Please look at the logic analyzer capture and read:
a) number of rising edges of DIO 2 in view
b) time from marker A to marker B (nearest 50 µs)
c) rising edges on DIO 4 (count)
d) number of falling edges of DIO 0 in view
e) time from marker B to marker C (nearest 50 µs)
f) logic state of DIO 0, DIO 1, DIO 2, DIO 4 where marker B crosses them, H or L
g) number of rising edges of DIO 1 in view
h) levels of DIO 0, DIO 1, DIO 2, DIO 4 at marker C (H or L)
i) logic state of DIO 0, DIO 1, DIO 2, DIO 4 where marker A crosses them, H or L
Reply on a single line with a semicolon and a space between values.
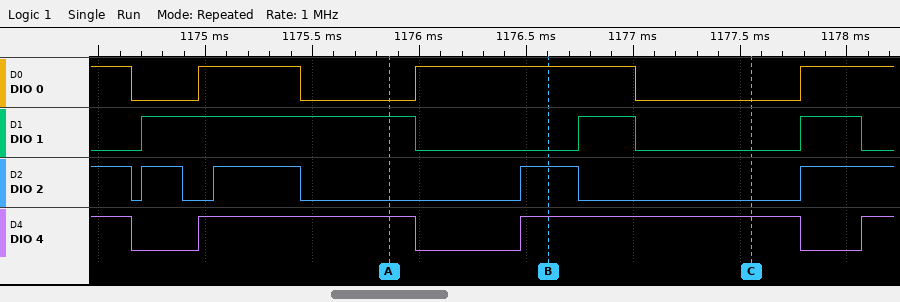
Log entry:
4; 750 µs; 3; 3; 950 µs; DIO 0=H, DIO 1=L, DIO 2=H, DIO 4=H; 3; DIO 0=L, DIO 1=L, DIO 2=L, DIO 4=H; DIO 0=L, DIO 1=H, DIO 2=L, DIO 4=H
